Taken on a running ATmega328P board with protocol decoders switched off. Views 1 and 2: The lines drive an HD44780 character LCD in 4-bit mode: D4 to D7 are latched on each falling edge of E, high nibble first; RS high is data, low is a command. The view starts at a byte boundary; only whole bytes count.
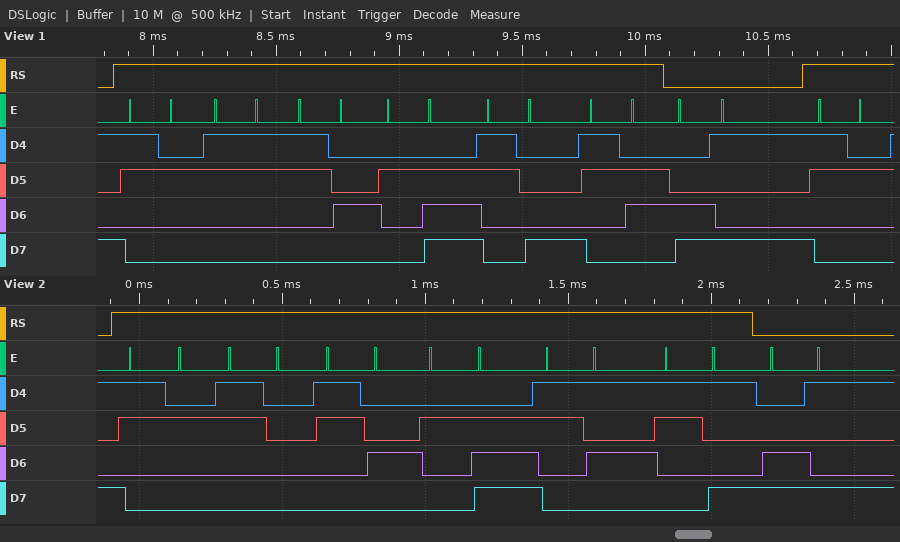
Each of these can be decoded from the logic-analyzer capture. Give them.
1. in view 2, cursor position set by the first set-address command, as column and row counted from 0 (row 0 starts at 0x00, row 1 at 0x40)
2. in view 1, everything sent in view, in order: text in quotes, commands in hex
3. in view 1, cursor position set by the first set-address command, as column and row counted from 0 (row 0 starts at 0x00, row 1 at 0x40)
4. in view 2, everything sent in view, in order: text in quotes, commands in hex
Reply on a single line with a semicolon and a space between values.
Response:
column 9, row 1; "234.86" 0xC9 "2"; column 9, row 1; "204.59" 0xC9
